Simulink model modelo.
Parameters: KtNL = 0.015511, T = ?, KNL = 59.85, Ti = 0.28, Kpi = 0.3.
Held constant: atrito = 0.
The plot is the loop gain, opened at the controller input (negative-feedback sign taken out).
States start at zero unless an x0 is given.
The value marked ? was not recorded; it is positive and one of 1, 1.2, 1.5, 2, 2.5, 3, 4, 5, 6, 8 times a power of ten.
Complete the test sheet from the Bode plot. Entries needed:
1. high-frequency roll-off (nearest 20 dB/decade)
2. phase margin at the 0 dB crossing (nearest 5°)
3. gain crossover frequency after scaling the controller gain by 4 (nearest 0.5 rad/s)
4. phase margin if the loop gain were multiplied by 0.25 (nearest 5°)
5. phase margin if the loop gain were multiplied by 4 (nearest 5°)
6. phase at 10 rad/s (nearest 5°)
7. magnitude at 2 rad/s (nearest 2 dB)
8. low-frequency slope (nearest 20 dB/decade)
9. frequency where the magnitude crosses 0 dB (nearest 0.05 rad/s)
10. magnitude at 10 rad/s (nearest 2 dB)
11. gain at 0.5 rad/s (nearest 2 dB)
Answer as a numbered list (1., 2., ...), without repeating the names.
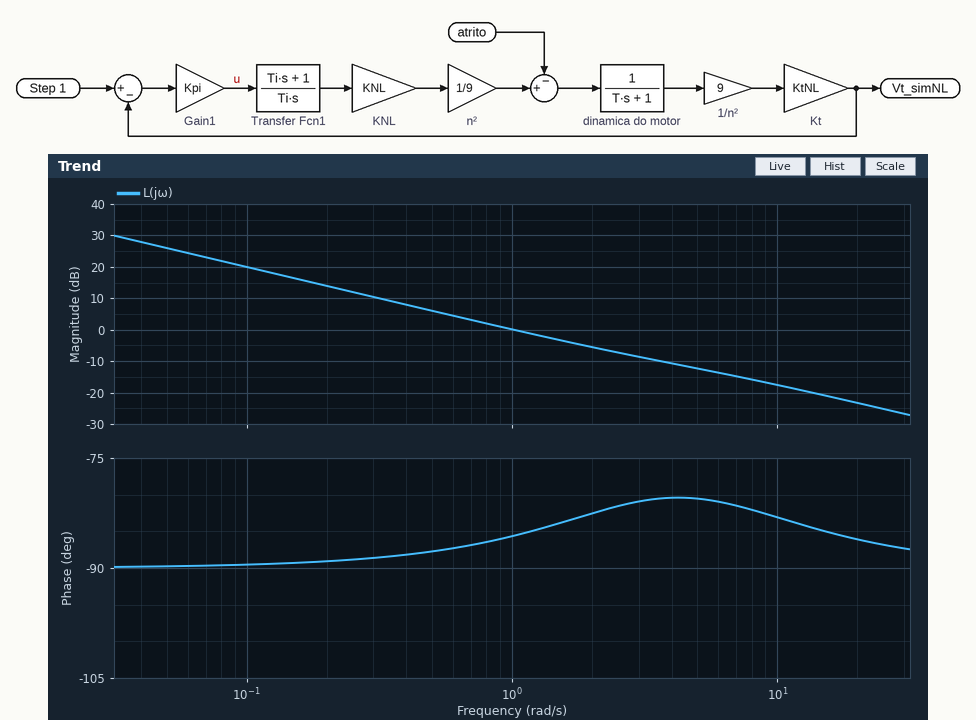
1. -20 dB/decade
2. 95°
3. 5.0 rad/s
4. 90°
5. 100°
6. -85°
7. -6 dB
8. -20 dB/decade
9. 1.00 rad/s
10. -18 dB
11. 6 dB
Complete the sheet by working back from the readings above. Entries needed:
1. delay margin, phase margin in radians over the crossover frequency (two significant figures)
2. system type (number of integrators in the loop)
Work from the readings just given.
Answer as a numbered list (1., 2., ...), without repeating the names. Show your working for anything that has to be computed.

1. 95 × π / 180 / 1 = 1.7 s
2. 1
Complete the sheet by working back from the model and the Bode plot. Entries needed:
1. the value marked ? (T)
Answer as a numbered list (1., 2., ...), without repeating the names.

1. 0.2
